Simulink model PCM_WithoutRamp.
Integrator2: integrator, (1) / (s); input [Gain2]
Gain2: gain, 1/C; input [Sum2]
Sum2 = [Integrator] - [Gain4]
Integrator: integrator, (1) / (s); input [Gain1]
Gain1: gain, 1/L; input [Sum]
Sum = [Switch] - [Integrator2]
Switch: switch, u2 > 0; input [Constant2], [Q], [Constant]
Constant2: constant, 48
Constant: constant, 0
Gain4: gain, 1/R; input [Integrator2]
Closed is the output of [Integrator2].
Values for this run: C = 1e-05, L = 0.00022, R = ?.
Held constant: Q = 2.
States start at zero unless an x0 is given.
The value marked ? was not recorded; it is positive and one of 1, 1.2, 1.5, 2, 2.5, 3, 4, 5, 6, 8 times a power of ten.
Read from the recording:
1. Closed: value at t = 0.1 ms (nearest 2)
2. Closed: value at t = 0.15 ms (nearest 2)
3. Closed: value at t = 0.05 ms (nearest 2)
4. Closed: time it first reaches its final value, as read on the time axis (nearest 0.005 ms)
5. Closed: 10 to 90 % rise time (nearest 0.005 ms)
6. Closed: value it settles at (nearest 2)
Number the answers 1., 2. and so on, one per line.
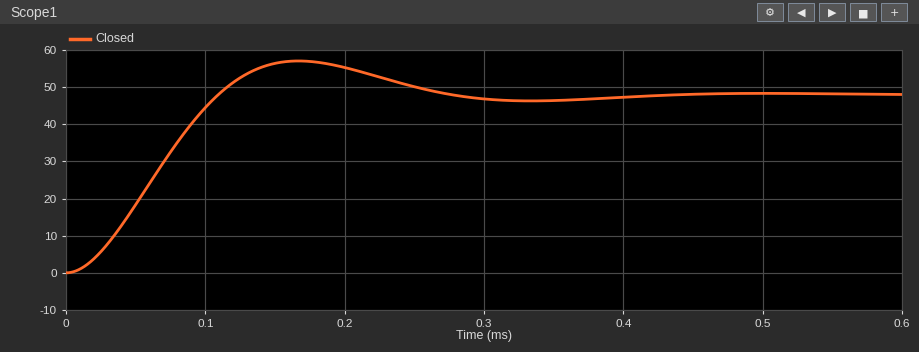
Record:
1. 44
2. 56
3. 18
4. 0.110 ms
5. 0.075 ms
6. 48
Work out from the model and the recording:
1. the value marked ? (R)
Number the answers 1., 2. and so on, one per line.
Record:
1. 5
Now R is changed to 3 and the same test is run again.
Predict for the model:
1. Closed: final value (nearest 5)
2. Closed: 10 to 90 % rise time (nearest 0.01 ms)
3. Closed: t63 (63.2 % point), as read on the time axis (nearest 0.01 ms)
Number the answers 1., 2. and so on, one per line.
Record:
1. 50
2. 0.11 ms
3. 0.09 ms
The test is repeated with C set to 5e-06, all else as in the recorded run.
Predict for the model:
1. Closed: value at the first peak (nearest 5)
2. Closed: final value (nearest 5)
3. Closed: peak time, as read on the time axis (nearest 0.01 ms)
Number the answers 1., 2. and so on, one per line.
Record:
1. 50
2. 50
3. 0.14 ms
